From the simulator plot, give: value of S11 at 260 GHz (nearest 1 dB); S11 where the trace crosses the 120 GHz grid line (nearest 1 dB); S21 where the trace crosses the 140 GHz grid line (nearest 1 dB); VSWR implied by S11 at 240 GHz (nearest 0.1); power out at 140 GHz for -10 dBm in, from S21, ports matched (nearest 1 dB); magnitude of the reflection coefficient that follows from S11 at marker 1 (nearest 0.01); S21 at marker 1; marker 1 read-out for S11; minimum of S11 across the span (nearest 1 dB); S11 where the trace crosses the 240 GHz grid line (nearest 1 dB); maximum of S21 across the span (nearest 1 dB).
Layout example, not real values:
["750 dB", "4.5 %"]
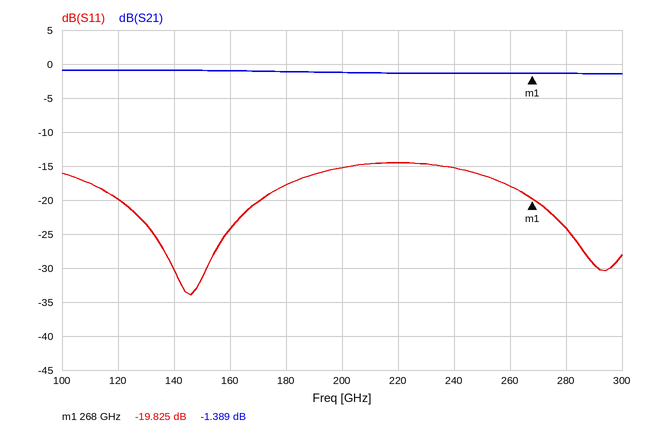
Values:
["-18 dB", "-20 dB", "-1 dB", "1.4", "-11 dBm", "0.10", "-1.389 dB", "-19.825 dB", "-34 dB", "-15 dB", "-1 dB"]
